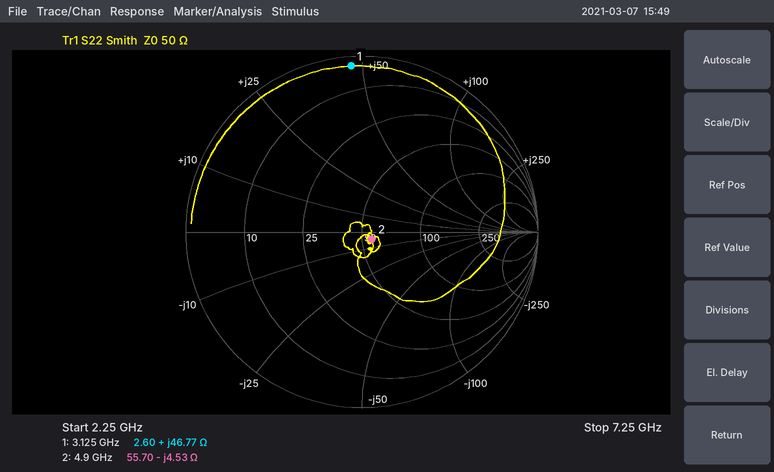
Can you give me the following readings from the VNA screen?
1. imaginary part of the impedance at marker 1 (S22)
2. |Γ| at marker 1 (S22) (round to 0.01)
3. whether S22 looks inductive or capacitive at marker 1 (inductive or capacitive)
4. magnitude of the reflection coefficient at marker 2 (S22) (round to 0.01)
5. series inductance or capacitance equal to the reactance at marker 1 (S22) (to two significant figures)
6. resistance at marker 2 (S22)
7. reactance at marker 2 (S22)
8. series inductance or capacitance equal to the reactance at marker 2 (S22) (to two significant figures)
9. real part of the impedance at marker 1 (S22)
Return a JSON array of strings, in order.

["+46.77 Ω", "0.95", "inductive", "0.07", "2.4 nH", "55.70 Ω", "-4.53 Ω", "7.2 pF", "2.60 Ω"]
